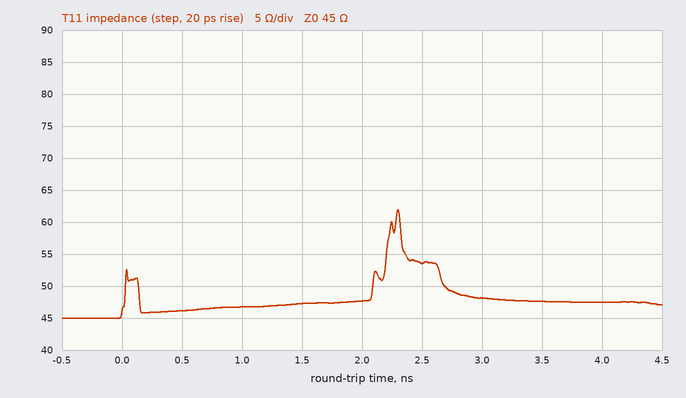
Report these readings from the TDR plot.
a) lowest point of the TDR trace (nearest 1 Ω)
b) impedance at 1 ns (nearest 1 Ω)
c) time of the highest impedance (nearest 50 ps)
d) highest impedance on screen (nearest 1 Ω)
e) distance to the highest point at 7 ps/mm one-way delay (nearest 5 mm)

45 Ω
47 Ω
2.30 ns
62 Ω
165 mm
